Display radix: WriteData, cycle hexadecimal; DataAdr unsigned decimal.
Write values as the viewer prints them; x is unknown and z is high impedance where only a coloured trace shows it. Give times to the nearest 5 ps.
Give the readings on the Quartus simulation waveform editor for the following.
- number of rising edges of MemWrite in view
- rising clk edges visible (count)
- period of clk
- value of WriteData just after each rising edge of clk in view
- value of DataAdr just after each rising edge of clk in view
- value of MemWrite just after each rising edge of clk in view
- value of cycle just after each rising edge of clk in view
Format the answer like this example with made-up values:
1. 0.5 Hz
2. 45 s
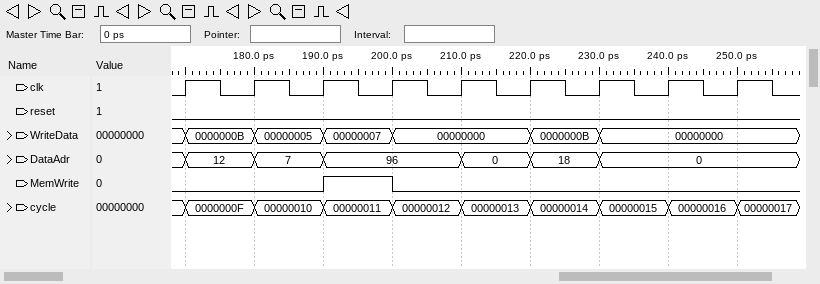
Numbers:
1. 1
2. 9
3. 10 ps
4. 0000000B, 00000005, 00000007, 00000000, 00000000, 0000000B, 00000000, 00000000, 00000000
5. 12, 7, 96, 96, 0, 18, 0, 0, 0
6. 0 0 1 0 0 0 0 0 0
7. 0000000F, 00000010, 00000011, 00000012, 00000013, 00000014, 00000015, 00000016, 00000017
